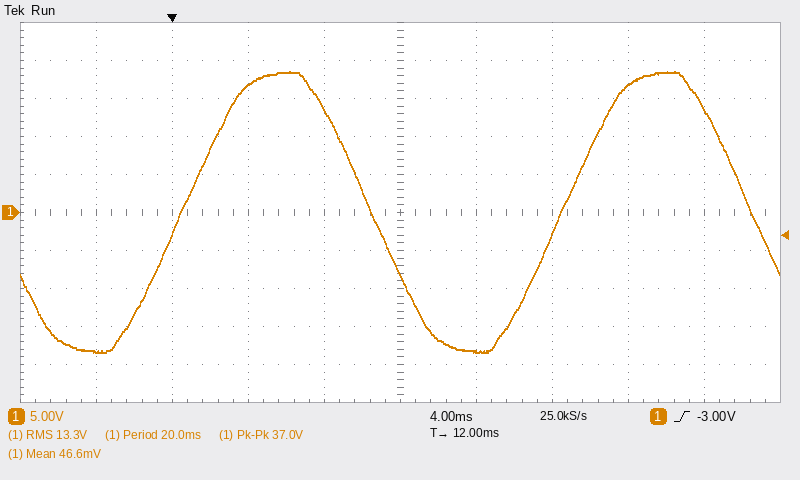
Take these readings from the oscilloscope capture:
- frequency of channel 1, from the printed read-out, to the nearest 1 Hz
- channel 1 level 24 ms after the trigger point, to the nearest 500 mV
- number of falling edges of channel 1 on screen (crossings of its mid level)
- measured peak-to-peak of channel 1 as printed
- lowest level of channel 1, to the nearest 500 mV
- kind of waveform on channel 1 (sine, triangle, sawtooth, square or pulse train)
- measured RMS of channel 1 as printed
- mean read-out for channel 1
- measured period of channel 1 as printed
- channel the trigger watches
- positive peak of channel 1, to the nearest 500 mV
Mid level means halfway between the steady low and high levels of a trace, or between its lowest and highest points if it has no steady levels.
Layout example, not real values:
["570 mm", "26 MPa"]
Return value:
["50 Hz", "16.5 V", "2", "37.0 V", "-18.5 V", "sine", "13.3 V", "46.6 mV", "20.0 ms", "channel 1", "18.5 V"]
